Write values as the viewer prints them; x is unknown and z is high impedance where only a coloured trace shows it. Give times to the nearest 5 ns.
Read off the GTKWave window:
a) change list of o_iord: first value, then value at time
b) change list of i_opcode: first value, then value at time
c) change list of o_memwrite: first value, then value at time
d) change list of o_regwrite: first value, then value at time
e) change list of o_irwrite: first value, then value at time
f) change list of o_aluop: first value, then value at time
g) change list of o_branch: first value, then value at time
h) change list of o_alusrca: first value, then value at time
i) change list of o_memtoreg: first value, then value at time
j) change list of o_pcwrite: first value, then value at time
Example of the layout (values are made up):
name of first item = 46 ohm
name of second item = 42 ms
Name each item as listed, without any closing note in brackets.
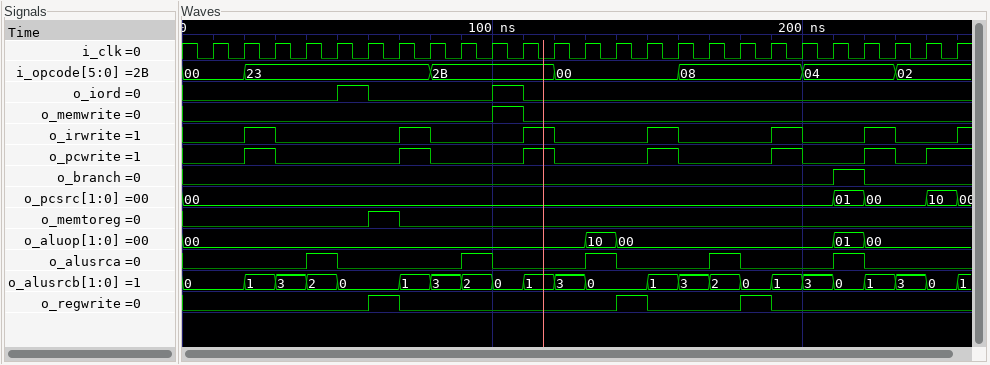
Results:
change list of o_iord: first value, then value at time = 0, 1 at 50 ns, 0 at 60 ns, 1 at 100 ns, 0 at 110 ns
change list of i_opcode: first value, then value at time = 00, 23 at 20 ns, 2B at 80 ns, 00 at 120 ns, 08 at 160 ns, 04 at 200 ns, 02 at 230 ns
change list of o_memwrite: first value, then value at time = 0, 1 at 100 ns, 0 at 110 ns
change list of o_regwrite: first value, then value at time = 0, 1 at 60 ns, 0 at 70 ns, 1 at 140 ns, 0 at 150 ns, 1 at 180 ns, 0 at 190 ns
change list of o_irwrite: first value, then value at time = 0, 1 at 20 ns, 0 at 30 ns, 1 at 70 ns, 0 at 80 ns, 1 at 110 ns, 0 at 120 ns, 1 at 150 ns, 0 at 160 ns, 1 at 190 ns, 0 at 200 ns, 1 at 220 ns, 0 at 230 ns, 1 at 250 ns
change list of o_aluop: first value, then value at time = 00, 10 at 130 ns, 00 at 140 ns, 01 at 210 ns, 00 at 220 ns
change list of o_branch: first value, then value at time = 0, 1 at 210 ns, 0 at 220 ns
change list of o_alusrca: first value, then value at time = 0, 1 at 40 ns, 0 at 50 ns, 1 at 90 ns, 0 at 100 ns, 1 at 130 ns, 0 at 140 ns, 1 at 170 ns, 0 at 180 ns, 1 at 210 ns, 0 at 220 ns
change list of o_memtoreg: first value, then value at time = 0, 1 at 60 ns, 0 at 70 ns
change list of o_pcwrite: first value, then value at time = 0, 1 at 20 ns, 0 at 30 ns, 1 at 70 ns, 0 at 80 ns, 1 at 110 ns, 0 at 120 ns, 1 at 150 ns, 0 at 160 ns, 1 at 190 ns, 0 at 200 ns, 1 at 220 ns, 0 at 230 ns, 1 at 240 ns
